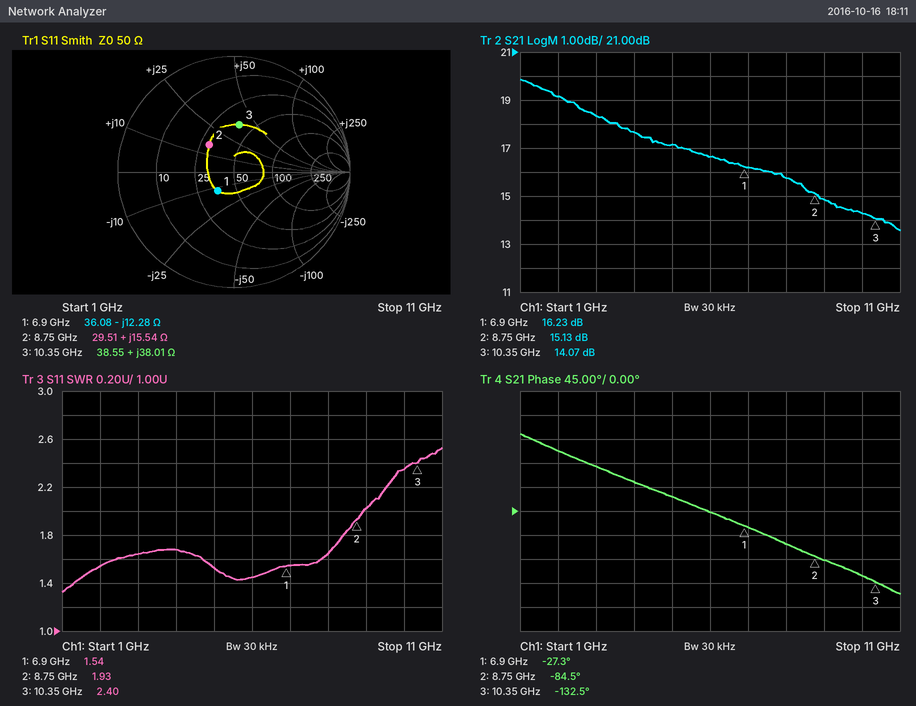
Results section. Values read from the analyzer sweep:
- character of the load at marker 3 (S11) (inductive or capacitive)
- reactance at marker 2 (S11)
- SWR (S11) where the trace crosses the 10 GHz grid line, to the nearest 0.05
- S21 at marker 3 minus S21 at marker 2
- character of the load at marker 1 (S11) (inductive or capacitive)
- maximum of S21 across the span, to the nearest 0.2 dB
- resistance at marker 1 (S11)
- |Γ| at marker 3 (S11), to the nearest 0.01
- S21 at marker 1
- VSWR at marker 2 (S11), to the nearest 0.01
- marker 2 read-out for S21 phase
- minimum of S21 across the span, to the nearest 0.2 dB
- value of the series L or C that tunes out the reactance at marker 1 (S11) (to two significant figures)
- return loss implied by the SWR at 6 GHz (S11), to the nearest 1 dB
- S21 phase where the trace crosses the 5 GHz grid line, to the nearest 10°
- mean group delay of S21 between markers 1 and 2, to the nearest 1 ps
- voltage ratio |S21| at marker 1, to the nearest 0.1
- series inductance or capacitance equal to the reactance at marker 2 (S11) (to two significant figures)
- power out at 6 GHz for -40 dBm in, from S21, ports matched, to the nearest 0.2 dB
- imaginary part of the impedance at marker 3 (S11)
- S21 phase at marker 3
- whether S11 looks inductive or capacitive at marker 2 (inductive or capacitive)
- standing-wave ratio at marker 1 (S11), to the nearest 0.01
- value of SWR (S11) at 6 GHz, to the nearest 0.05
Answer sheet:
inductive
+15.54 Ω
2.35
-1.06 dB
capacitive
19.8 dB
36.08 Ω
0.41
16.23 dB
1.93
-84.5°
13.6 dB
280 pH
15 dB
30°
86 ps
6.5
280 pH
-23.4 dBm
+38.01 Ω
-132.5°
inductive
1.54
1.45
